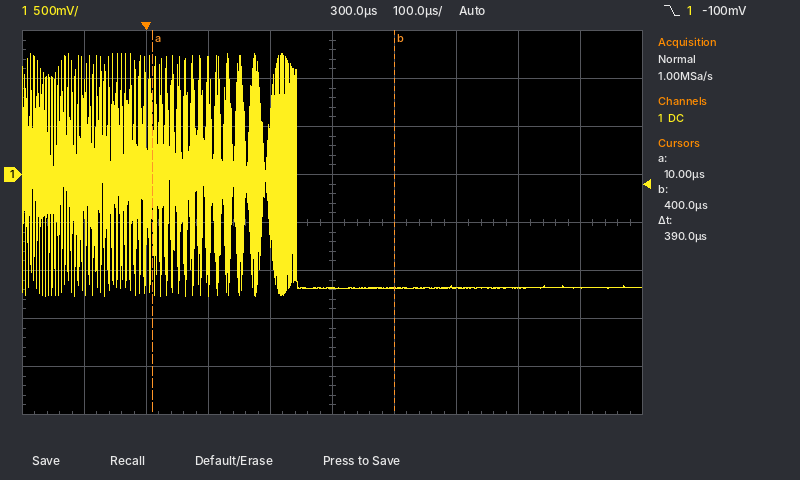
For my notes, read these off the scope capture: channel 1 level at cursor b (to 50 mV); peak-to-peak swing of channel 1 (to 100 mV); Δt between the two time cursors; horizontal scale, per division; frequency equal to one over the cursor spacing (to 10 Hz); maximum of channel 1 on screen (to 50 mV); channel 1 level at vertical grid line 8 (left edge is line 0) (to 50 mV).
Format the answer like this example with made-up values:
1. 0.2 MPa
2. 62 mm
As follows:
1. -1.20 V
2. 2.50 V
3. 390 µs
4. 100 µs
5. 2.56 kHz
6. 1.25 V
7. -1.20 V
